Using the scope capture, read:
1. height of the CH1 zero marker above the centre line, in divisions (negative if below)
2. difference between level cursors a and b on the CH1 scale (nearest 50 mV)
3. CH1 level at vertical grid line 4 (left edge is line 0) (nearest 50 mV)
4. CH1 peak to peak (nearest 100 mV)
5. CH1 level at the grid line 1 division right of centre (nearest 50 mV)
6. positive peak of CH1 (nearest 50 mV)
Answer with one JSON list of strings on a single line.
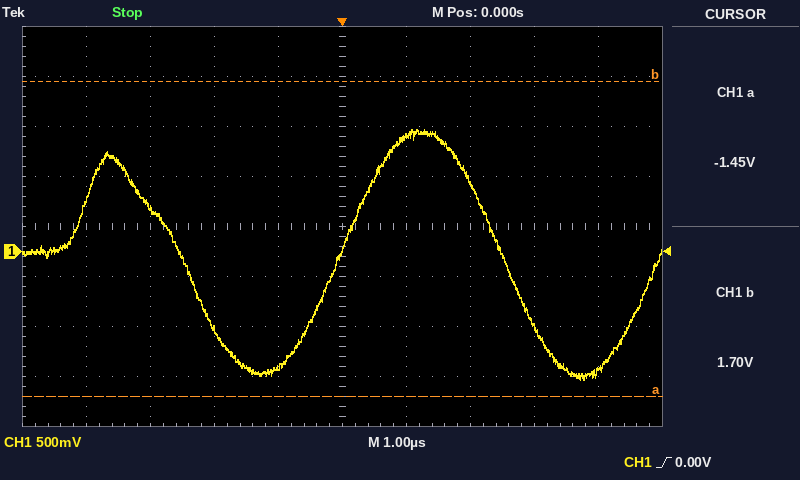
["-0.5 div", "3.15 V", "-1.15 V", "2.50 V", "1.15 V", "1.20 V"]
